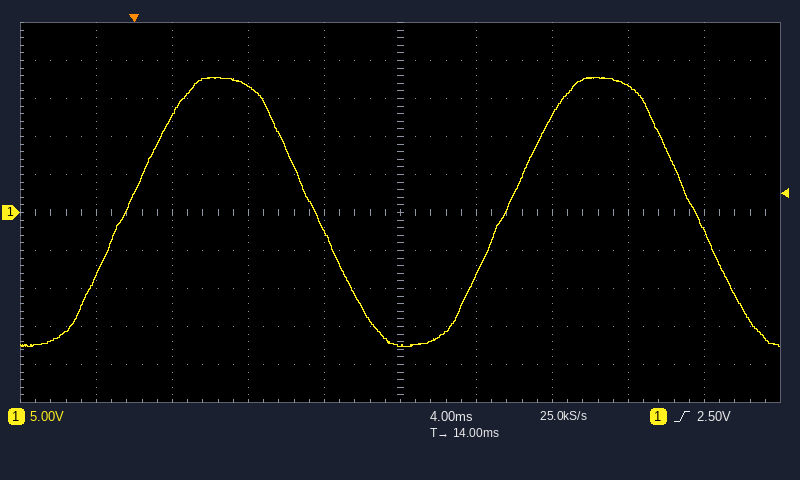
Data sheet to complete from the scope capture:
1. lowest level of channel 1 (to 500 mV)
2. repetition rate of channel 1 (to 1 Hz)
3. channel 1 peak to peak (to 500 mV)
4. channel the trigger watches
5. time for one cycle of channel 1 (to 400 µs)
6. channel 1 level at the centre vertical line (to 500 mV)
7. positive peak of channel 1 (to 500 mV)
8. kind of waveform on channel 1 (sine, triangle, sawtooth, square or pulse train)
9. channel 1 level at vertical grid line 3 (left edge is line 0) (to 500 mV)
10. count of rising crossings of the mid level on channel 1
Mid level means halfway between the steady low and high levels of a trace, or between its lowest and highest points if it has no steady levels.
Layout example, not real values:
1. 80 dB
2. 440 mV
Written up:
1. -17.5 V
2. 50 Hz
3. 35.5 V
4. channel 1
5. 20.0 ms
6. -17.5 V
7. 18.0 V
8. sine
9. 16.5 V
10. 2
